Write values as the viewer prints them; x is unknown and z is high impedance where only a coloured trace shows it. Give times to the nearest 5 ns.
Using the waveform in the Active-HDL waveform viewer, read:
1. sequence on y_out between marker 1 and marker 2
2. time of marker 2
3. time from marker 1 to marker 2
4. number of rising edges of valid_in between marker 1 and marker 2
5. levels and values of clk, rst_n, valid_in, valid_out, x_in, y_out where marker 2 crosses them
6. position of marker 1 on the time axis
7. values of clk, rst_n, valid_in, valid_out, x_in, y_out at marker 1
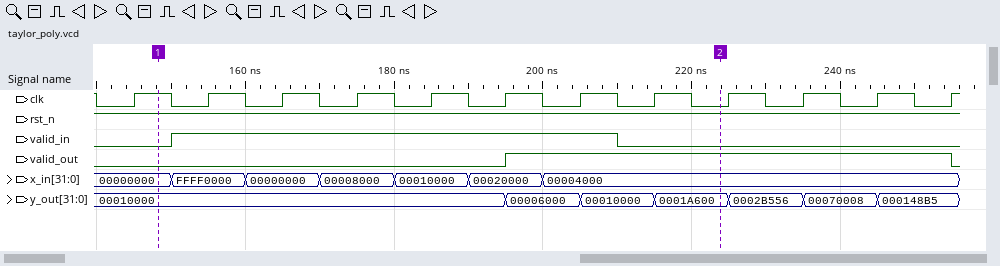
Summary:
00010000, 00006000, 00010000, 0001A600
225 ns
75 ns
1
clk=0, rst_n=1, valid_in=0, valid_out=1, x_in=00004000, y_out=0001A600
150 ns
clk=1, rst_n=1, valid_in=0, valid_out=0, x_in=00000000, y_out=00010000
